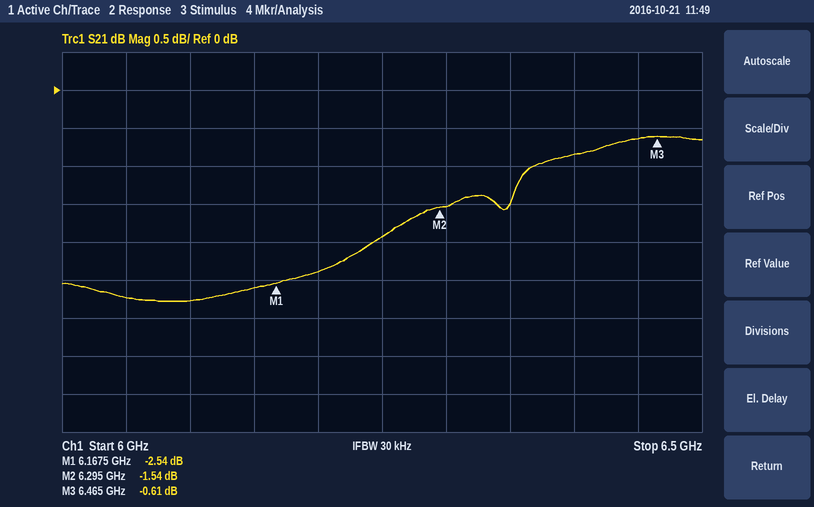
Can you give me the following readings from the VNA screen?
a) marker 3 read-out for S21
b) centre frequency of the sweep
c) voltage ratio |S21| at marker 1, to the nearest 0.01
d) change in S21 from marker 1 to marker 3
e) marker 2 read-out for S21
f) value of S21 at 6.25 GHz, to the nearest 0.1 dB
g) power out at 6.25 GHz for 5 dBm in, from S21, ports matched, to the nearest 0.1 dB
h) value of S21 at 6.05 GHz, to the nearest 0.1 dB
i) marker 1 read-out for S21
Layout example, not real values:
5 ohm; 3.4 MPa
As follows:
-0.61 dB; 6.25 GHz; 0.75; 1.93 dB; -1.54 dB; -1.9 dB; 3.1 dBm; -2.7 dB; -2.54 dB
